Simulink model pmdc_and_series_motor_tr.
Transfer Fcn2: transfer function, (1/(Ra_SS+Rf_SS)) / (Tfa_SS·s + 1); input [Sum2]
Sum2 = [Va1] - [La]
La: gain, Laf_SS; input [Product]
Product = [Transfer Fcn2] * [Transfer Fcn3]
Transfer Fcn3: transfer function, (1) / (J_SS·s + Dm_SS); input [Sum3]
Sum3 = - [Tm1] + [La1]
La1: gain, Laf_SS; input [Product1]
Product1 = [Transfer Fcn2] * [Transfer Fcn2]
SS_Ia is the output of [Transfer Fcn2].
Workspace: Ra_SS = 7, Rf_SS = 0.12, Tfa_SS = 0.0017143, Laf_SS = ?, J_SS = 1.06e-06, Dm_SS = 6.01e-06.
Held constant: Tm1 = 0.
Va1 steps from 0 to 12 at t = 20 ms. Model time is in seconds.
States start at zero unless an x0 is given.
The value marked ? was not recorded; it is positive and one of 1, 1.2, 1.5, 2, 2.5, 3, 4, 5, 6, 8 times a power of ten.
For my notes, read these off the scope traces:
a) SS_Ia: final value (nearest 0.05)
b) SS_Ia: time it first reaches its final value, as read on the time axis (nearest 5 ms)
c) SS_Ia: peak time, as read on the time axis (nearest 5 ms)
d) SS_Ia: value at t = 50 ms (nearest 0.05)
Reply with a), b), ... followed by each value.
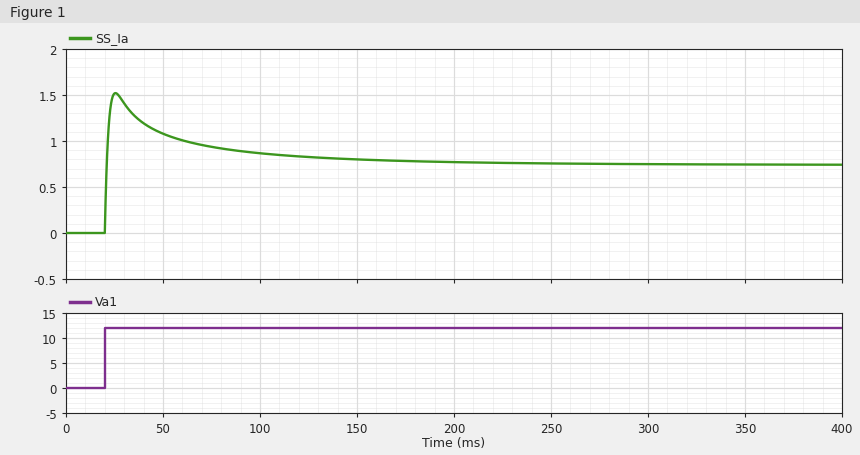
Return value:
a) 0.75
b) 20 ms
c) 25 ms
d) 1.10
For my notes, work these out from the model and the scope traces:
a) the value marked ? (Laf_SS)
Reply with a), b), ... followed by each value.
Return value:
a) 0.01
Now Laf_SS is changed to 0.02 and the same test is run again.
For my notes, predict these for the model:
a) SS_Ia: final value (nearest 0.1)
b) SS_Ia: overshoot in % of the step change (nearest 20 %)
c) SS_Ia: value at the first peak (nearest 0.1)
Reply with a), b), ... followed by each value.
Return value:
a) 0.5
b) 180 %
c) 1.4
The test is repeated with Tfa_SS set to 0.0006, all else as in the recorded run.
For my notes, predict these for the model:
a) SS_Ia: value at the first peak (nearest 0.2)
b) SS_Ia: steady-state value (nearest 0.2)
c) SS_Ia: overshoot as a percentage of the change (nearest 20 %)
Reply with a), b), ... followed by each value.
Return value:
a) 1.6
b) 0.8
c) 120 %
